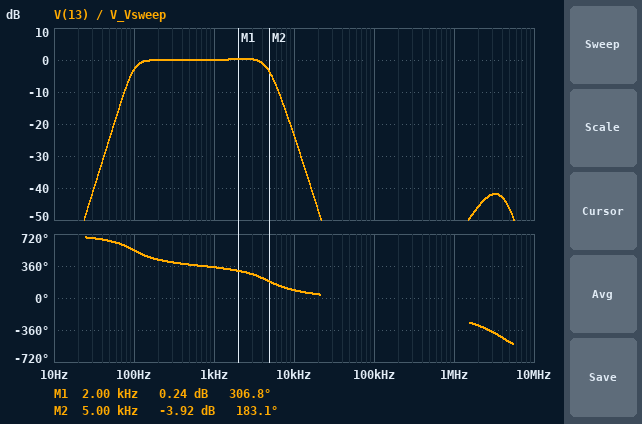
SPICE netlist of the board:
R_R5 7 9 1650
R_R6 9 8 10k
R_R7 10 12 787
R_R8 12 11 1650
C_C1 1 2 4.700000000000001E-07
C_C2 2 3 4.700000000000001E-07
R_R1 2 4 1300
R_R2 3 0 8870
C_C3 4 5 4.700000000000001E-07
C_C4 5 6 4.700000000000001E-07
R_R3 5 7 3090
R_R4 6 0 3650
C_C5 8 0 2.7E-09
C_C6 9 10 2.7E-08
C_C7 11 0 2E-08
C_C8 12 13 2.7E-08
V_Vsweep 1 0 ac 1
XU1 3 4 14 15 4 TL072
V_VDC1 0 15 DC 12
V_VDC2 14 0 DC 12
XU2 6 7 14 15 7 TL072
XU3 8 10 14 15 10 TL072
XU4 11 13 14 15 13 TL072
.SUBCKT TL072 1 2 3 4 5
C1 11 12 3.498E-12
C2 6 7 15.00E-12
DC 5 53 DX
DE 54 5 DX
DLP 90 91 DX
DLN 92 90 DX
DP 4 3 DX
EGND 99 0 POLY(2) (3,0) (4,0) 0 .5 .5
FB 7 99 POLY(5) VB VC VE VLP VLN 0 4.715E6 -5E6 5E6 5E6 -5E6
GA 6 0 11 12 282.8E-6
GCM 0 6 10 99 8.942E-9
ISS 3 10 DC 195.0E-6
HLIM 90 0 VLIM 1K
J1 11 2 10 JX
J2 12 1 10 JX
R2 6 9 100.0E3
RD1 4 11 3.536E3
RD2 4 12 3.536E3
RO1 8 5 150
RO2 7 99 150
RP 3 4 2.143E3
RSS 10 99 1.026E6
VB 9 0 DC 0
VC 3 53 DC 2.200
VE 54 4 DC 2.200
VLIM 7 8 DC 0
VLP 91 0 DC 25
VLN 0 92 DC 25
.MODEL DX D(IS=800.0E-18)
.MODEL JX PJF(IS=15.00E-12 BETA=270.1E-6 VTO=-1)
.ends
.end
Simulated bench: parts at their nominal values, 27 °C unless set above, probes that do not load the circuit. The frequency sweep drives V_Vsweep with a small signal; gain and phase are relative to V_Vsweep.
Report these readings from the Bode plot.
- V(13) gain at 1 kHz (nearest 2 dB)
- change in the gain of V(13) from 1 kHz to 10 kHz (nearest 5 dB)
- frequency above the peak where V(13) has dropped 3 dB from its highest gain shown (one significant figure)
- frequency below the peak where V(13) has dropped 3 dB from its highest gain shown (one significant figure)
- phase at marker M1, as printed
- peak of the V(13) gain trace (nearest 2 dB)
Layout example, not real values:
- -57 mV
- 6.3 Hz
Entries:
- 0 dB
- -25 dB
- 5 kHz
- 100 Hz
- 306.8 deg
- 0 dB
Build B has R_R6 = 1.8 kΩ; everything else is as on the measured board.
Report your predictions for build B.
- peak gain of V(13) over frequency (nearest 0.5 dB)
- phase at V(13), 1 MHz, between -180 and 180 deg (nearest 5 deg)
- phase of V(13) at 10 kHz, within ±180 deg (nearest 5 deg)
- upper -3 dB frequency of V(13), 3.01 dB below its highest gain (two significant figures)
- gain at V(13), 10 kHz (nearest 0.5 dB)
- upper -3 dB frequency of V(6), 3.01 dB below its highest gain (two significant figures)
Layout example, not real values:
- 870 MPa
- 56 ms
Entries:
- 0 dB
- 115 deg
- 165 deg
- 6.0 kHz
- -6.5 dB
- 3.8 MHz
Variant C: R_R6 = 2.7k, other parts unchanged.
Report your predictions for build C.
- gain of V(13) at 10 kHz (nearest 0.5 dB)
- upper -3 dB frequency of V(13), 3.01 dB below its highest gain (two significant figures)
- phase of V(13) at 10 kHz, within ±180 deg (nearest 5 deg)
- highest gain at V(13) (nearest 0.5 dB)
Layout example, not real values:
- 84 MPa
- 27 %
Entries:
- -9.0 dB
- 7.3 kHz
- 130 deg
- 0 dB
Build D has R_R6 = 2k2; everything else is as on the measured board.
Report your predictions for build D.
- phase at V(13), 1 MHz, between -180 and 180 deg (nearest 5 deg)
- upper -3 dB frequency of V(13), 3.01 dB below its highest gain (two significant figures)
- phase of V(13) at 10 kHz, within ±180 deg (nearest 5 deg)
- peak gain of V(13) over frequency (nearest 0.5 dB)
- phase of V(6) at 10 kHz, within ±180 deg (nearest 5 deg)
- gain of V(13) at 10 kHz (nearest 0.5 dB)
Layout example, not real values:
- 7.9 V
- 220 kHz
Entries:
- 115 deg
- 6.7 kHz
- 145 deg
- 0 dB
- 0 deg
- -7.5 dB
